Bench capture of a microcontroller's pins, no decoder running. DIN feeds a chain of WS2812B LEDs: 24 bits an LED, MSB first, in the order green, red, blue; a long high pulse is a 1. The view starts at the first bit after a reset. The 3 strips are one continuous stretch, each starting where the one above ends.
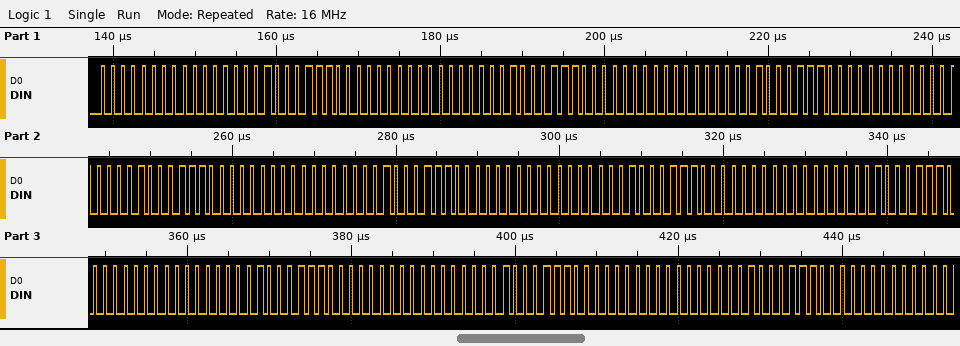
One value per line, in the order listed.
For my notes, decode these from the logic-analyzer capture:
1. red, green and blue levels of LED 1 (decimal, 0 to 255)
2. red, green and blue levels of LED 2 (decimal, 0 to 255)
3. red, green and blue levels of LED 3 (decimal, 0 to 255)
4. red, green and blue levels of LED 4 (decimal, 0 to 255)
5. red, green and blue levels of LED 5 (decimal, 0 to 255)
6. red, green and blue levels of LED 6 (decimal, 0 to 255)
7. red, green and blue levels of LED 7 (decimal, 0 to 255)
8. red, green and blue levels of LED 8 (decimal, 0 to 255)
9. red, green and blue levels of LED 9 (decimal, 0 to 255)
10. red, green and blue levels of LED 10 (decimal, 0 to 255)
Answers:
0, 0, 142
0, 0, 142
0, 0, 142
0, 0, 142
0, 0, 142
0, 0, 142
0, 0, 142
0, 0, 142
0, 0, 142
0, 0, 142
